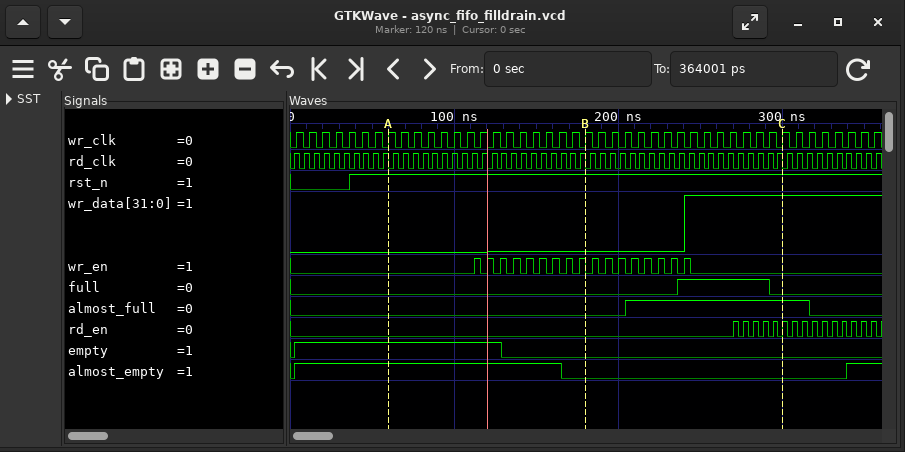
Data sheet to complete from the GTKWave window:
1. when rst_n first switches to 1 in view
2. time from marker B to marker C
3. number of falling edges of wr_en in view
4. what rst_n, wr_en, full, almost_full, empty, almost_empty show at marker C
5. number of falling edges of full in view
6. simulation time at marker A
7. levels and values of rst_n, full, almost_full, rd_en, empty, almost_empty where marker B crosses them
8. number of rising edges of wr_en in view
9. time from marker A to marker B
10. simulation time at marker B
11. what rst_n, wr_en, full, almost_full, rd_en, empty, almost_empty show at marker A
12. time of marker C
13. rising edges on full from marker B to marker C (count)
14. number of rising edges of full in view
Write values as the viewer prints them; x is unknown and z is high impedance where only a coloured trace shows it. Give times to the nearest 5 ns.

35 ns
120 ns
17
rst_n=1, wr_en=0, full=0, almost_full=1, empty=0, almost_empty=0
1
60 ns
rst_n=1, full=0, almost_full=0, rd_en=0, empty=0, almost_empty=0
17
120 ns
180 ns
rst_n=1, wr_en=0, full=0, almost_full=0, rd_en=0, empty=1, almost_empty=1
300 ns
1
1
